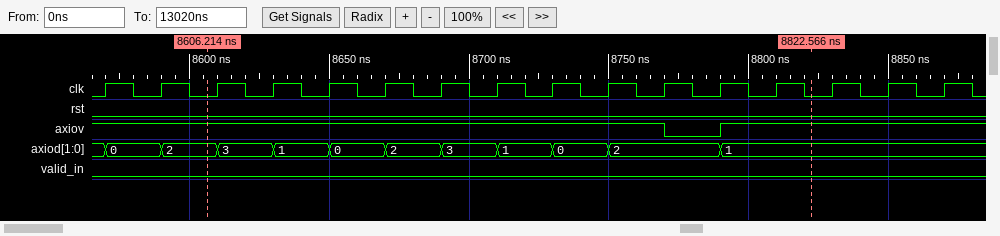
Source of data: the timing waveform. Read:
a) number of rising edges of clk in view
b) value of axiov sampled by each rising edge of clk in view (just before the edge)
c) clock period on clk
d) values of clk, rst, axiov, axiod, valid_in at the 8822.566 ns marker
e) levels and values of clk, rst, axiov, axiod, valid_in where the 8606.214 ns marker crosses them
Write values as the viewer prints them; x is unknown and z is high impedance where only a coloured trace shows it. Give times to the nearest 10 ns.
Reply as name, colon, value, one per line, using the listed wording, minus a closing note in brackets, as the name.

number of rising edges of clk in view: 16
value of axiov sampled by each rising edge of clk in view: 1 1 1 1 1 1 1 1 1 1 1 0 1 1 1 1
clock period on clk: 20 ns
values of clk, rst, axiov, axiod, valid_in at the 8822.566 ns marker: clk=0, rst=0, axiov=1, axiod=1, valid_in=0
levels and values of clk, rst, axiov, axiod, valid_in where the 8606.214 ns marker crosses them: clk=0, rst=0, axiov=1, axiod=2, valid_in=0
